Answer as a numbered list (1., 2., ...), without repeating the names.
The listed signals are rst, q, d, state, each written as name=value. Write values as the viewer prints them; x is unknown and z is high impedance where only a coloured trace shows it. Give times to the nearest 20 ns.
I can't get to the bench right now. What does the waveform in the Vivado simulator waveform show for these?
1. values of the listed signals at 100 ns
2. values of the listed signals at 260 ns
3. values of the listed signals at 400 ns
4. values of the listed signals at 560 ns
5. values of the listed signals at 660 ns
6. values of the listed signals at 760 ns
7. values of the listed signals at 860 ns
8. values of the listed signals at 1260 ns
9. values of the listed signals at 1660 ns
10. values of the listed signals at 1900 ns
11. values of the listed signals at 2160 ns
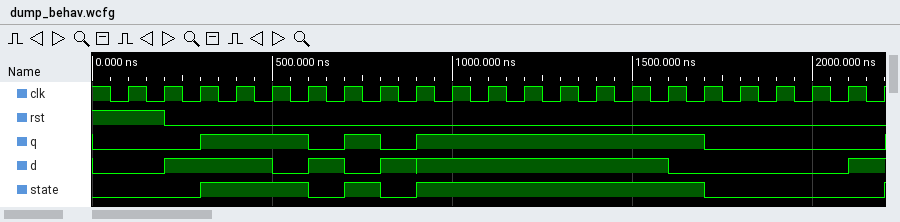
1. rst=1, q=0, d=0, state=0
2. rst=0, q=0, d=1, state=0
3. rst=0, q=1, d=1, state=1
4. rst=0, q=1, d=0, state=1
5. rst=0, q=0, d=1, state=0
6. rst=0, q=1, d=0, state=1
7. rst=0, q=0, d=1, state=0
8. rst=0, q=1, d=1, state=1
9. rst=0, q=1, d=0, state=1
10. rst=0, q=0, d=0, state=0
11. rst=0, q=0, d=1, state=0
